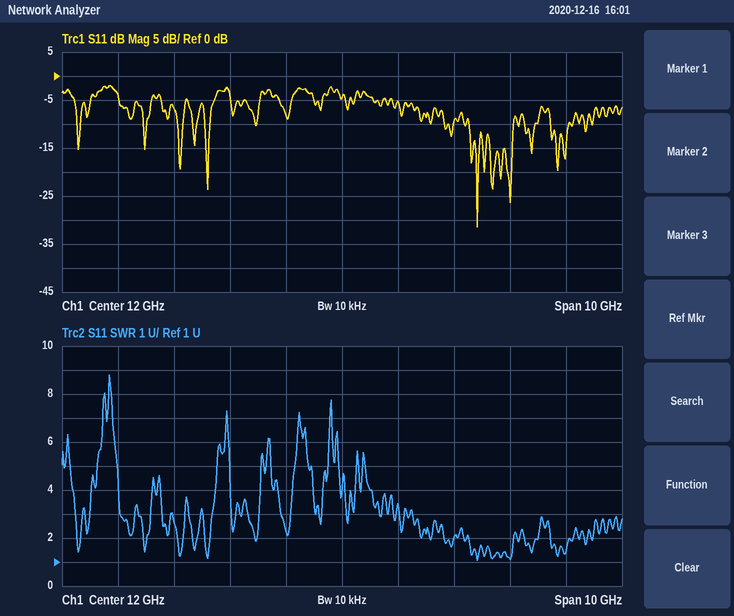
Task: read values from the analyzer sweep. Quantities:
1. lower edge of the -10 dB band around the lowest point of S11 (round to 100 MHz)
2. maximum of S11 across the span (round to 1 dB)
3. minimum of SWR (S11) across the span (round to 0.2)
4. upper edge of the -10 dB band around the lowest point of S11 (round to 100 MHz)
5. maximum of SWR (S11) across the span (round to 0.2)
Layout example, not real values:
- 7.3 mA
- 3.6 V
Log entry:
- 14.3 GHz
- -2 dB
- 1.0
- 15.1 GHz
- 8.8
